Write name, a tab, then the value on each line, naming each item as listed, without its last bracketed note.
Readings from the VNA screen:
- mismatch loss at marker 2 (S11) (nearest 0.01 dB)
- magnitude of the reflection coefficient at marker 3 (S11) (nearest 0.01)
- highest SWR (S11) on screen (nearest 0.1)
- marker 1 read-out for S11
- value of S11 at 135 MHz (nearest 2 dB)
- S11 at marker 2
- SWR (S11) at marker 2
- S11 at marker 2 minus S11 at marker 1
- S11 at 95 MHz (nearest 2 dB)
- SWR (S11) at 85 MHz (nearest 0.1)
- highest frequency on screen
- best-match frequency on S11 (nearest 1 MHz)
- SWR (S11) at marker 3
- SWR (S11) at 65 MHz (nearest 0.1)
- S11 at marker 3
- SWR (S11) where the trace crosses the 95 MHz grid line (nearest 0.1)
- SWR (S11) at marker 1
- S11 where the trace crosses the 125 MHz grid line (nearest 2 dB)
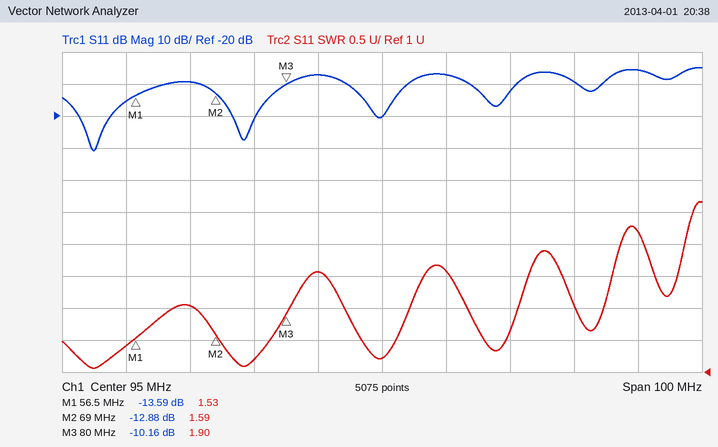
mismatch loss at marker 2 (S11)	0.23 dB
magnitude of the reflection coefficient at marker 3 (S11)	0.31
highest SWR (S11) on screen	3.7
marker 1 read-out for S11	-13.59 dB
value of S11 at 135 MHz	-6 dB
S11 at marker 2	-12.88 dB
SWR (S11) at marker 2	1.59
S11 at marker 2 minus S11 at marker 1	0.71 dB
S11 at 95 MHz	-20 dB
SWR (S11) at 85 MHz	2.6
highest frequency on screen	145 MHz
best-match frequency on S11	50 MHz
SWR (S11) at marker 3	1.90
SWR (S11) at 65 MHz	2.0
S11 at marker 3	-10.16 dB
SWR (S11) where the trace crosses the 95 MHz grid line	1.2
SWR (S11) at marker 1	1.53
S11 where the trace crosses the 125 MHz grid line	-10 dB
